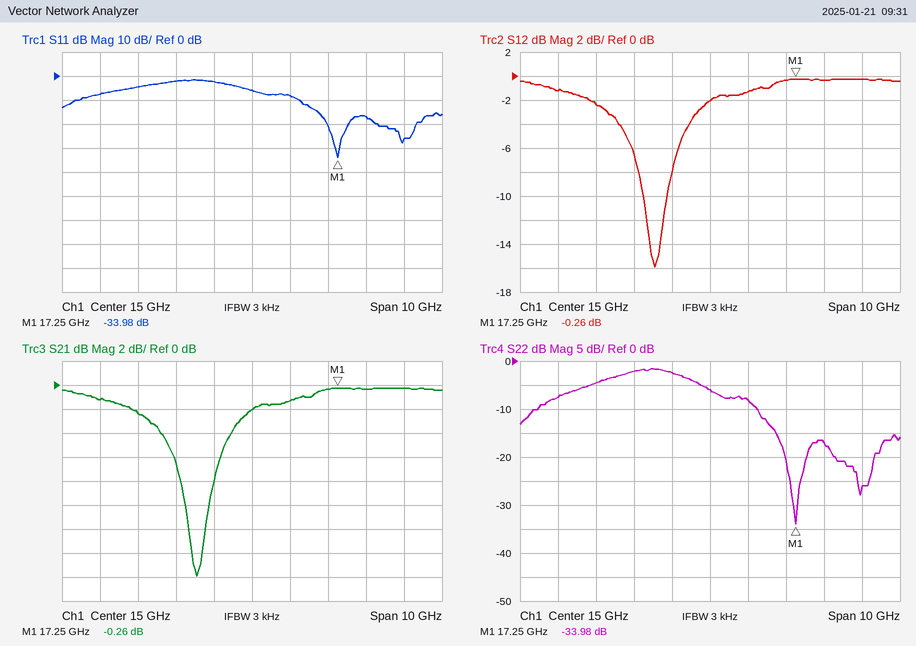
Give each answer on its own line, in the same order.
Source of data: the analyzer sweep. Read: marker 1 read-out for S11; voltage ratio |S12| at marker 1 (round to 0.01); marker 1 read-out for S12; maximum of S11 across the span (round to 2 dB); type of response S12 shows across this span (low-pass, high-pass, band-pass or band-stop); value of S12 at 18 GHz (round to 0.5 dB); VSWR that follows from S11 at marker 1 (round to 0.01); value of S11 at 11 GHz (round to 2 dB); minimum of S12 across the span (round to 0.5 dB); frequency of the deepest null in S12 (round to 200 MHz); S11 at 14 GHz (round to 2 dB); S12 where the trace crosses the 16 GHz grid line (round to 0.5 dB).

-33.98 dB
0.97
-0.26 dB
-2 dB
band-stop
-0.5 dB
1.04
-8 dB
-16.0 dB
13.6 GHz
-2 dB
-1.5 dB
